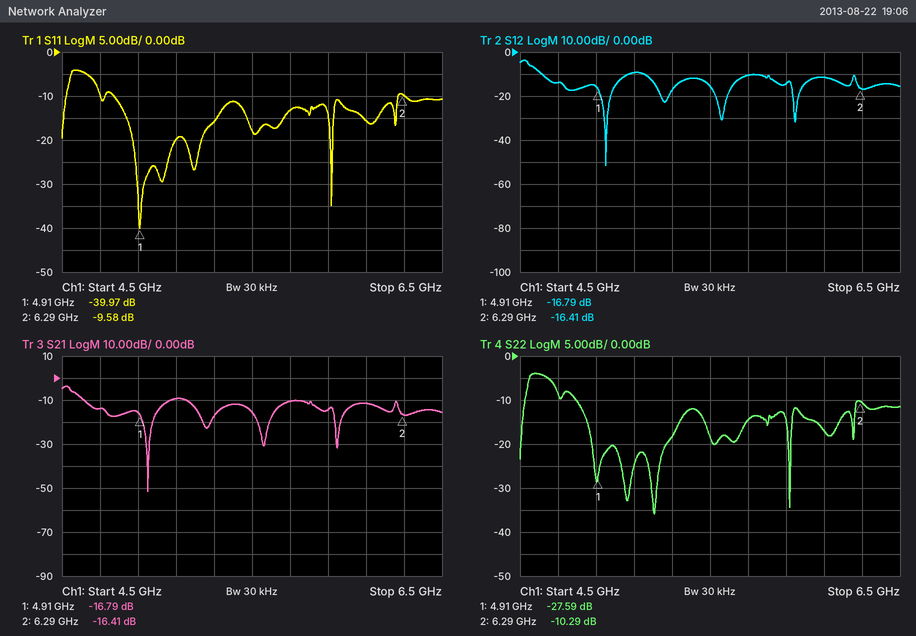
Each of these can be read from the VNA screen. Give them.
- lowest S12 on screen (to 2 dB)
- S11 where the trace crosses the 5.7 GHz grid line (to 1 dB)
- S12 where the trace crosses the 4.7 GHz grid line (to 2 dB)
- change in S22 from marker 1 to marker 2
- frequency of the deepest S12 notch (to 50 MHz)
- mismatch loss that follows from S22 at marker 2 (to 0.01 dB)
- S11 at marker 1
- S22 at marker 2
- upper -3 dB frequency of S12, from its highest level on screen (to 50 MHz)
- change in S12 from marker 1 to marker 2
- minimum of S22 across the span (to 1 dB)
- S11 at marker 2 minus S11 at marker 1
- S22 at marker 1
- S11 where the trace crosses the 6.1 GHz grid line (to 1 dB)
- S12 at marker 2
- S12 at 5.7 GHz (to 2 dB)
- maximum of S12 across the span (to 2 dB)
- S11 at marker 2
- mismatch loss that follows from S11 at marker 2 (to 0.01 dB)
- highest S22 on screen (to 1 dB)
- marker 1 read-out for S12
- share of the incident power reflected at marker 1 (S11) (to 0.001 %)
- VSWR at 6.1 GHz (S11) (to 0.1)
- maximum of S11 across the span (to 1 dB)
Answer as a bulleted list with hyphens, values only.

- -52 dB
- -13 dB
- -14 dB
- 17.30 dB
- 4.95 GHz
- 0.43 dB
- -39.97 dB
- -10.29 dB
- 4.55 GHz
- 0.38 dB
- -36 dB
- 30.39 dB
- -27.59 dB
- -16 dB
- -16.41 dB
- -10 dB
- -4 dB
- -9.58 dB
- 0.51 dB
- -4 dB
- -16.79 dB
- 0.010 %
- 1.4
- -4 dB
